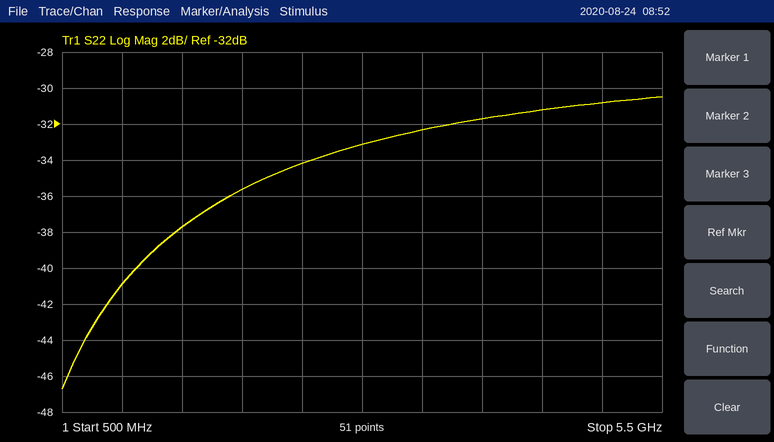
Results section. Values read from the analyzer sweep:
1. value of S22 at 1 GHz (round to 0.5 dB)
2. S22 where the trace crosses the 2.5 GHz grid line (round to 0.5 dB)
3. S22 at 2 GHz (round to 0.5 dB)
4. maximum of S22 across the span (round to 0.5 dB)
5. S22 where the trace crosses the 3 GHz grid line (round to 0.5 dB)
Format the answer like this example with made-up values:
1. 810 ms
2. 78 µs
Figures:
1. -41.0 dB
2. -34.0 dB
3. -35.5 dB
4. -30.5 dB
5. -33.0 dB
